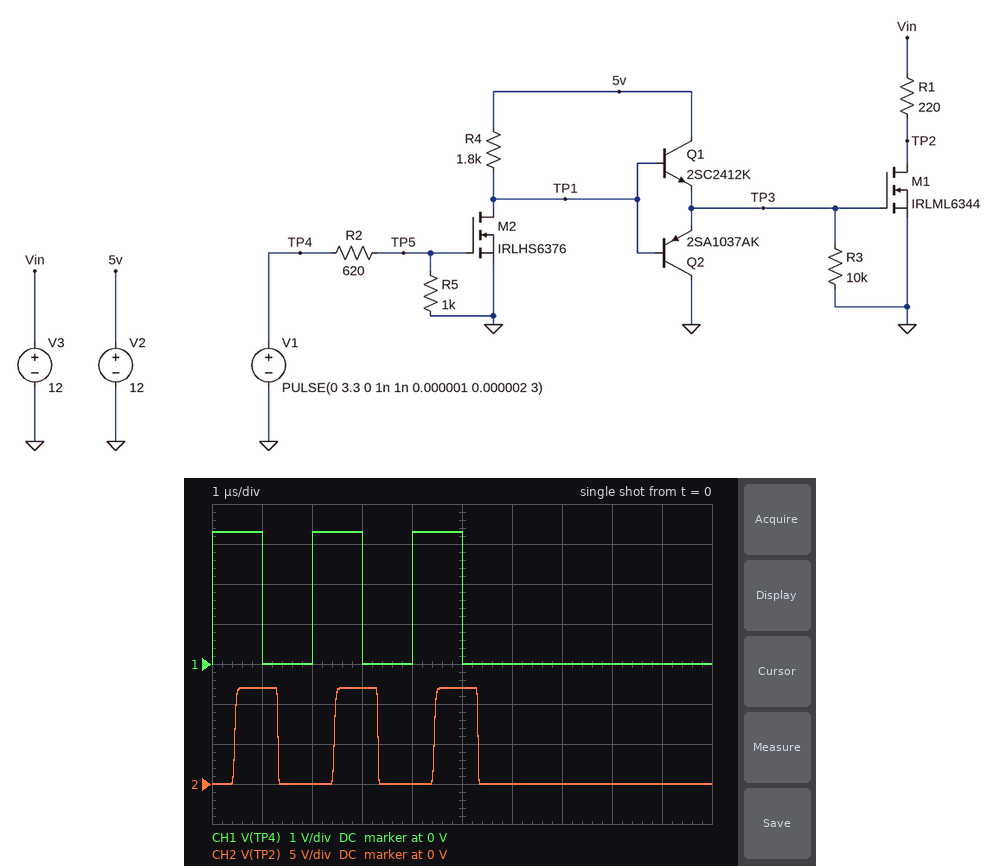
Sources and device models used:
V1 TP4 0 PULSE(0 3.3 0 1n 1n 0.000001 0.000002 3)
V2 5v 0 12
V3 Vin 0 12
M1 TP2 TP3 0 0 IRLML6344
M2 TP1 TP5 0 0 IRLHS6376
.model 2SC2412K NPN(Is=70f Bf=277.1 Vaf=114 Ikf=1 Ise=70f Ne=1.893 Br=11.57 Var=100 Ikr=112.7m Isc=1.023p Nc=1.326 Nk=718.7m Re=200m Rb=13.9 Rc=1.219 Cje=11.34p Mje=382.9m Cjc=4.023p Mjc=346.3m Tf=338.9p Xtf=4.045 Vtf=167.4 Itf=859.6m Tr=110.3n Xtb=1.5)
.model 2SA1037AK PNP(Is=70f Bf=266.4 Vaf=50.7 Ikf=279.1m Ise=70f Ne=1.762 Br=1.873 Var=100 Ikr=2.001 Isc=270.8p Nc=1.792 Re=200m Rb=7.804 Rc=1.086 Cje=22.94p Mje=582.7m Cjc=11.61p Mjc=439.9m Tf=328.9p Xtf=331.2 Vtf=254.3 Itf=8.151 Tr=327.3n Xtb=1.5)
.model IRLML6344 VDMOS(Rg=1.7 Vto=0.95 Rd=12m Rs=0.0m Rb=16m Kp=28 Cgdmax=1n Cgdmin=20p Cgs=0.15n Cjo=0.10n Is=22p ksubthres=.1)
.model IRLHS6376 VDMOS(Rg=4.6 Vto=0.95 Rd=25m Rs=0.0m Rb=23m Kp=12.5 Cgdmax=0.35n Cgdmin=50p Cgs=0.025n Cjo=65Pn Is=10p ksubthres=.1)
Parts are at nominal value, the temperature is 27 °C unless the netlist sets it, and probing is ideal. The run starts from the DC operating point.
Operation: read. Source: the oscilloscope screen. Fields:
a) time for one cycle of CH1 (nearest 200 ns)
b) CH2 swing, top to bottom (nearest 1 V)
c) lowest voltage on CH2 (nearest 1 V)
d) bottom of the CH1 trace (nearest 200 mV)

2.0 µs
12 V
0 V
0 V
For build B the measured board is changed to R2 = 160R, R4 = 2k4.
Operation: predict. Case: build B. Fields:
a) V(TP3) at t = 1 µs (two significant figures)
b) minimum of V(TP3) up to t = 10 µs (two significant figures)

390 mV
380 mV
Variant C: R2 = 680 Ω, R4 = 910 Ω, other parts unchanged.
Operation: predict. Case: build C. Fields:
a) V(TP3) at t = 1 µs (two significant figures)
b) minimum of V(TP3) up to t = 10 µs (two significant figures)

460 mV
440 mV
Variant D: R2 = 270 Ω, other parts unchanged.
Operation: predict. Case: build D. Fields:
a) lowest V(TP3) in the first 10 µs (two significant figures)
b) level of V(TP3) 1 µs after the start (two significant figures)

390 mV
400 mV
